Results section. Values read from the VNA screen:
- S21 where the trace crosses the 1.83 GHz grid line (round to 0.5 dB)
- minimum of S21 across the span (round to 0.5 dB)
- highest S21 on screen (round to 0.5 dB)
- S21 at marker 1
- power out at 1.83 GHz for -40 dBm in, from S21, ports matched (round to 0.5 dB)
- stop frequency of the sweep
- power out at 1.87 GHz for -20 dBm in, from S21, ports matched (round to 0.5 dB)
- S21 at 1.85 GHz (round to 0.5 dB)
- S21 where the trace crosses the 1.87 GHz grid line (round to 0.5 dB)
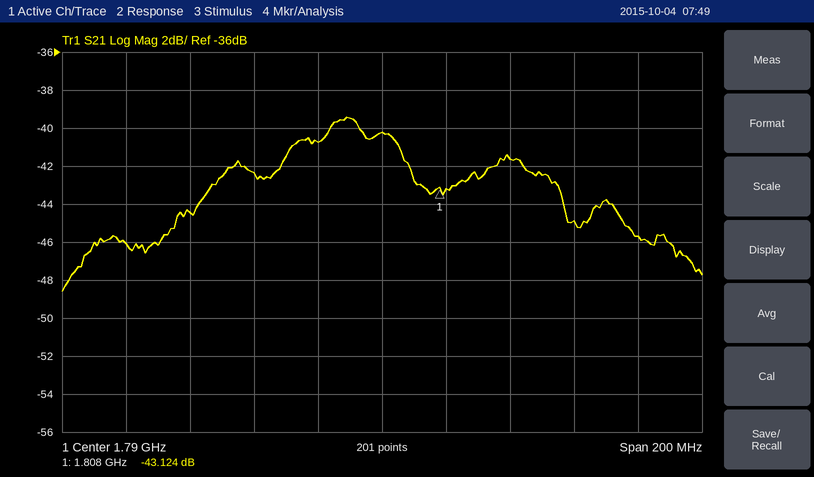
-41.5 dB
-48.5 dB
-39.5 dB
-43.124 dB
-81.5 dBm
1.89 GHz
-65.5 dBm
-45.0 dB
-45.5 dB
